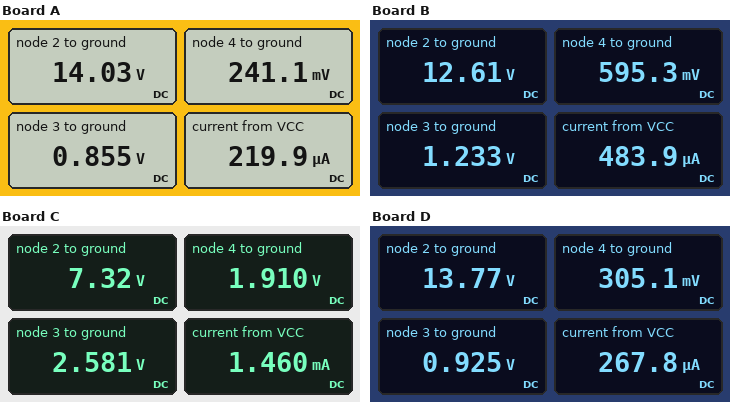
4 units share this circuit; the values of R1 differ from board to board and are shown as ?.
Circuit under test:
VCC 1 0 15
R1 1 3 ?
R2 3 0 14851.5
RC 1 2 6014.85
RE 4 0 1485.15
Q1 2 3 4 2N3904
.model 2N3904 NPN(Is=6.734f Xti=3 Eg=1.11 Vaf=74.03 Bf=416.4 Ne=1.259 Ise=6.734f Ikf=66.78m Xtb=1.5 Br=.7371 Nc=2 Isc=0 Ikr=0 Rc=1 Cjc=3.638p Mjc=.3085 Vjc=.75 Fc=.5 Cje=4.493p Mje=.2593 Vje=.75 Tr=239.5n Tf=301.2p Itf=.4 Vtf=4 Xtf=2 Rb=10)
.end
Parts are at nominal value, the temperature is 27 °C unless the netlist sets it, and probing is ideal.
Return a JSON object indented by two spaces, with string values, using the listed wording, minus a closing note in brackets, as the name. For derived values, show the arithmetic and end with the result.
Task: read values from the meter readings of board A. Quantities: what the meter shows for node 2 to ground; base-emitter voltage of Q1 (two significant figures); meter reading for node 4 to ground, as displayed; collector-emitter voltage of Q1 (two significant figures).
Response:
{
  "what the meter shows for node 2 to ground": "14.03 V",
  "base-emitter voltage of Q1": "855 mV - 241.1 mV = 610 mV",
  "meter reading for node 4 to ground, as displayed": "241.1 mV",
  "collector-emitter voltage of Q1": "14.03 V - 241.1 mV = 14 V"
}
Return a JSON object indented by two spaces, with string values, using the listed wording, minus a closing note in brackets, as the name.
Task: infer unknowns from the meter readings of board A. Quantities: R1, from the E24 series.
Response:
{
  "R1, from the E24 series": "240 kΩ"
}
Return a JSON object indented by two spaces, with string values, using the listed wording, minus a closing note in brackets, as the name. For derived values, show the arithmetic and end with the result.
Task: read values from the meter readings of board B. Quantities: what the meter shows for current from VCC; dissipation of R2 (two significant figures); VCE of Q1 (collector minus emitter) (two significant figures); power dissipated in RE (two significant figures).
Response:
{
  "what the meter shows for current from VCC": "483.9 µA",
  "dissipation of R2": "(1.233 V)^2 / 14.85 kΩ = 100 µW",
  "VCE of Q1 (collector minus emitter)": "12.61 V - 595.3 mV = 12 V",
  "power dissipated in RE": "(595.3 mV)^2 / 1.485 kΩ = 240 µW"
}
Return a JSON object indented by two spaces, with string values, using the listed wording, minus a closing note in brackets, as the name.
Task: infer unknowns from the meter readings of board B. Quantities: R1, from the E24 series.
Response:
{
  "R1, from the E24 series": "160 kΩ"
}
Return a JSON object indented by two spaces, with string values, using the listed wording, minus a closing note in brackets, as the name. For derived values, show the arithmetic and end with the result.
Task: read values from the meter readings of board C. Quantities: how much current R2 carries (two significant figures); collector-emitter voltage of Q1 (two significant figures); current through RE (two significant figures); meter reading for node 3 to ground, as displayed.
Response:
{
  "how much current R2 carries": "(2.581 V) / 14.85 kΩ = 170 µA",
  "collector-emitter voltage of Q1": "7.32 V - 1.91 V = 5.4 V",
  "current through RE": "(1.91 V) / 1.485 kΩ = 1.3 mA",
  "meter reading for node 3 to ground, as displayed": "2.581 V"
}
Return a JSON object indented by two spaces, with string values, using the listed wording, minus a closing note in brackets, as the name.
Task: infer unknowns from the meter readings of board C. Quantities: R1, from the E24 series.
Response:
{
  "R1, from the E24 series": "68 kΩ"
}
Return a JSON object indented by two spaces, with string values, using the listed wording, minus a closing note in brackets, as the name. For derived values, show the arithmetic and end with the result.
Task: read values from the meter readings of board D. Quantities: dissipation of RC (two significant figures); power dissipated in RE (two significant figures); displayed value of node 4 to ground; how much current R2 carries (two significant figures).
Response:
{
  "dissipation of RC": "(15 V - 13.77 V)^2 / 6.015 kΩ = 250 µW",
  "power dissipated in RE": "(305.1 mV)^2 / 1.485 kΩ = 63 µW",
  "displayed value of node 4 to ground": "305.1 mV",
  "how much current R2 carries": "(925 mV) / 14.85 kΩ = 62 µA"
}
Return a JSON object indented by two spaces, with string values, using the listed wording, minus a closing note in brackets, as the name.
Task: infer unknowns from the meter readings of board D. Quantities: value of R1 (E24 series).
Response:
{
  "value of R1": "220 kΩ"
}
